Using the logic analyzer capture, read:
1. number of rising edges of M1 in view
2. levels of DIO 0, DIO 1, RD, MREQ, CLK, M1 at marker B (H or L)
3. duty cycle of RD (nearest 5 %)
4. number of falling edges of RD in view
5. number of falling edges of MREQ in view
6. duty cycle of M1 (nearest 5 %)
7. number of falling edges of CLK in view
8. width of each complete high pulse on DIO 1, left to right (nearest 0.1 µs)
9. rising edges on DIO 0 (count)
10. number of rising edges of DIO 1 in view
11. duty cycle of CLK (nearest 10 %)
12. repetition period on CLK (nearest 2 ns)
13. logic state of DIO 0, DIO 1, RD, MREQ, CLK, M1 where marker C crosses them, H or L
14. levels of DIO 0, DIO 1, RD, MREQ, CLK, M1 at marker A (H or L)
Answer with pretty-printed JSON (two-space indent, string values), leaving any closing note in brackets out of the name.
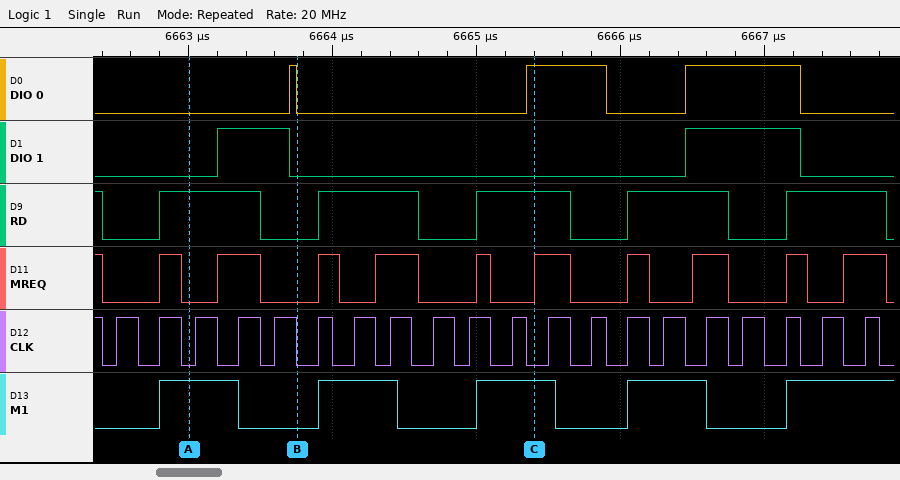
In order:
{
  "number of rising edges of M1 in view": "5",
  "levels of DIO 0, DIO 1, RD, MREQ, CLK, M1 at marker B": "DIO 0=L, DIO 1=L, RD=L, MREQ=L, CLK=L, M1=L",
  "duty cycle of RD": "65 %",
  "number of falling edges of RD in view": "6",
  "number of falling edges of MREQ in view": "11",
  "duty cycle of M1": "50 %",
  "number of falling edges of CLK in view": "21",
  "width of each complete high pulse on DIO 1, left to right": "0.5 µs, 0.8 µs",
  "rising edges on DIO 0": "3",
  "number of rising edges of DIO 1 in view": "2",
  "duty cycle of CLK": "50 %",
  "repetition period on CLK": "274 ns",
  "logic state of DIO 0, DIO 1, RD, MREQ, CLK, M1 where marker C crosses them, H or L": "DIO 0=H, DIO 1=L, RD=H, MREQ=H, CLK=L, M1=H",
  "levels of DIO 0, DIO 1, RD, MREQ, CLK, M1 at marker A": "DIO 0=L, DIO 1=L, RD=H, MREQ=L, CLK=L, M1=H"
}
